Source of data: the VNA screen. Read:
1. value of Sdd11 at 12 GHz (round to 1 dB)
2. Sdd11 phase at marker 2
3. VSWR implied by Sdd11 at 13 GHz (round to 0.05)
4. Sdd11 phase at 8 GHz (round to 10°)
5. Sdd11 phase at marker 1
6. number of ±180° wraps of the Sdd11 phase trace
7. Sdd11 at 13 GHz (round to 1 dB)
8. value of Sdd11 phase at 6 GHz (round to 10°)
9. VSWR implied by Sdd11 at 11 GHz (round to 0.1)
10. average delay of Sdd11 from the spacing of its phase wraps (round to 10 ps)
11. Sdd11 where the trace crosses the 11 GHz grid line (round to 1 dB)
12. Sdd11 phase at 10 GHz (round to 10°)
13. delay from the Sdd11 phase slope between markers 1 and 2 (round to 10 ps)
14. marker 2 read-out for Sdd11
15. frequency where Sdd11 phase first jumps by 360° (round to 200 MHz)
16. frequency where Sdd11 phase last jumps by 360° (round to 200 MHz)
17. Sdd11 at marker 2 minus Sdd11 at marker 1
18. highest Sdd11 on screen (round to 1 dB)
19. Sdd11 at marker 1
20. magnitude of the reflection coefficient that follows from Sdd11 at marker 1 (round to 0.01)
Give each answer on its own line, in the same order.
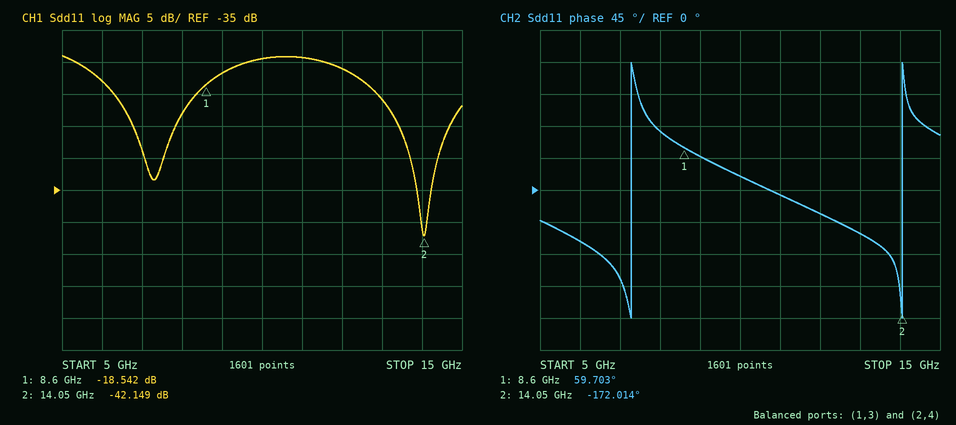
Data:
-16 dB
-172.014°
1.20
80°
59.703°
2
-21 dB
-70°
1.5
150 ps
-14 dB
20°
120 ps
-42.149 dB
7.2 GHz
14.0 GHz
-23.607 dB
-14 dB
-18.542 dB
0.12
